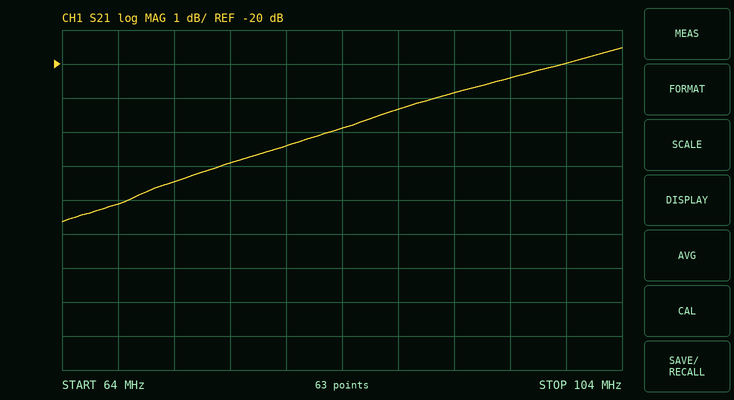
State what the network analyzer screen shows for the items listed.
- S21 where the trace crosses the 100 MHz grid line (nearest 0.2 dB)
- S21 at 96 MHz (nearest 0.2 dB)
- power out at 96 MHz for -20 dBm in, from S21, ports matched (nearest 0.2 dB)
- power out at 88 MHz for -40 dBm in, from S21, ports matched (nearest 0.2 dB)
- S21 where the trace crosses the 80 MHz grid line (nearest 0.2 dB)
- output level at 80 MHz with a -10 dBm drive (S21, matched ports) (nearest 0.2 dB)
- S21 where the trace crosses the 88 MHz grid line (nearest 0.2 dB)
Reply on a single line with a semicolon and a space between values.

-20.0 dB; -20.4 dB; -40.4 dBm; -61.4 dBm; -22.4 dB; -32.4 dBm; -21.4 dB
